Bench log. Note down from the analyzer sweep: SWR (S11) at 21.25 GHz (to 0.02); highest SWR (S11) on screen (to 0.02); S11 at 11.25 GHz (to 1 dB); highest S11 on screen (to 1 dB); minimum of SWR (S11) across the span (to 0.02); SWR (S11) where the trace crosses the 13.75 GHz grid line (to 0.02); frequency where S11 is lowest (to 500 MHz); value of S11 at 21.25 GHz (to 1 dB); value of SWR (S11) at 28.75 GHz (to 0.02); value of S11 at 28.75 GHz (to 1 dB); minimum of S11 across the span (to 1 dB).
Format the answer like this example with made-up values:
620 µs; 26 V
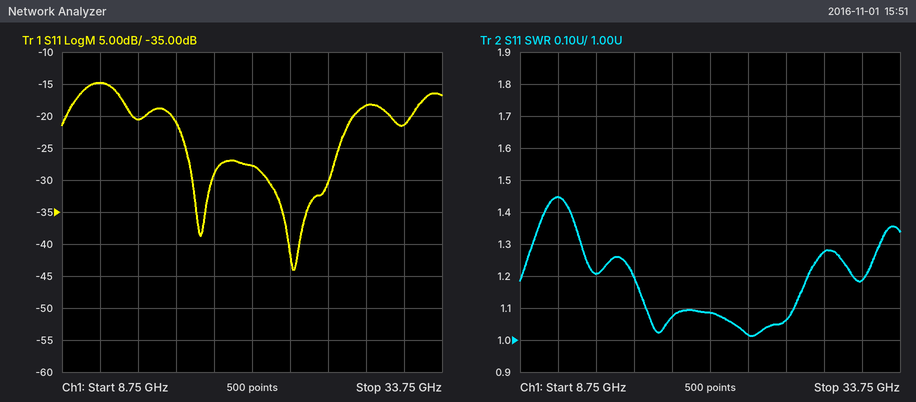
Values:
1.08; 1.44; -15 dB; -15 dB; 1.02; 1.20; 24.0 GHz; -28 dB; 1.28; -18 dB; -44 dB
